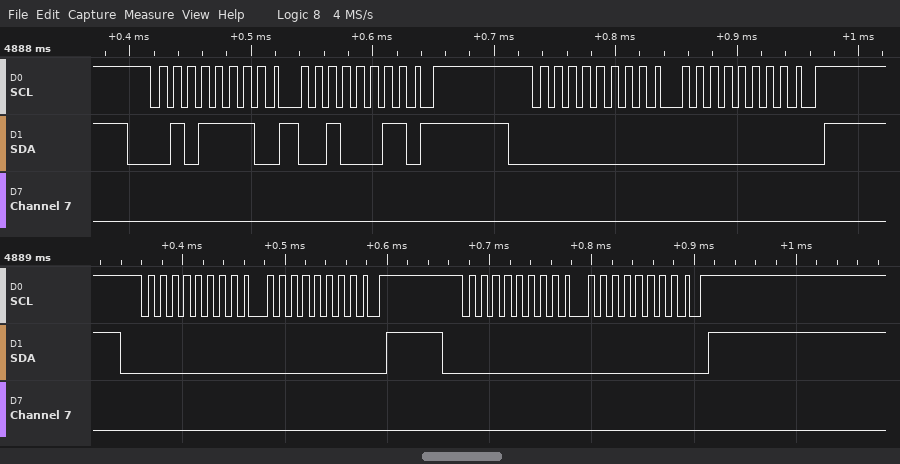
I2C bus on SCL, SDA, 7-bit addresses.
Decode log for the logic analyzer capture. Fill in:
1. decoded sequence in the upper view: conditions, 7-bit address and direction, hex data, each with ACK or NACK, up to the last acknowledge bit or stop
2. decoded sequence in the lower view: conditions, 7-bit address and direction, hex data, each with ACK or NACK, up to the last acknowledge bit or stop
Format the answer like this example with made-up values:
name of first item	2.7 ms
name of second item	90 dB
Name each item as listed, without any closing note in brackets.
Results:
decoded sequence in the upper view: conditions, 7-bit address and direction, hex data, each with ACK or NACK, up to the last acknowledge bit or stop	start, address 2F write ACK, 23 ACK, repeated start, address 00 write ACK, 00 ACK, stop
decoded sequence in the lower view: conditions, 7-bit address and direction, hex data, each with ACK or NACK, up to the last acknowledge bit or stop	start, address 00 write ACK, 00 ACK, stop, start, address 00 write ACK, 00 ACK, stop
